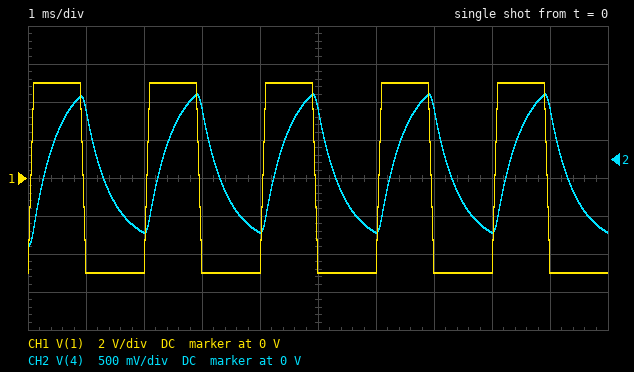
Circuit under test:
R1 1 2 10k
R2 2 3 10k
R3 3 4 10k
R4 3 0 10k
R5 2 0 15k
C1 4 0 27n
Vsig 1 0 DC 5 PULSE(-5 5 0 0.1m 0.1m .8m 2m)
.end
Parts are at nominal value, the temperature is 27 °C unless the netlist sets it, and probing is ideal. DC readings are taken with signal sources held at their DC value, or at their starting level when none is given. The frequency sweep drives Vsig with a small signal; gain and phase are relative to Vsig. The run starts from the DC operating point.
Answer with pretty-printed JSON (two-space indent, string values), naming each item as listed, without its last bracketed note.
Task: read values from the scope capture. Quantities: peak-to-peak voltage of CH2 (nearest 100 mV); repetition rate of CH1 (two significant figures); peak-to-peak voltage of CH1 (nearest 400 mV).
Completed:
{
  "peak-to-peak voltage of CH2": "2.0 V",
  "repetition rate of CH1": "500 Hz",
  "peak-to-peak voltage of CH1": "10.0 V"
}
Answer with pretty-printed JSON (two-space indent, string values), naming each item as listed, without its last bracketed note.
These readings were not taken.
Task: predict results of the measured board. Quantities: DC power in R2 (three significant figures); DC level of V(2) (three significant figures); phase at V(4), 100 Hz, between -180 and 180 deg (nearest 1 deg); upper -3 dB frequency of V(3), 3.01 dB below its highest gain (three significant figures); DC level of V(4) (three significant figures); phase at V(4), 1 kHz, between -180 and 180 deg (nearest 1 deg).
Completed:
{
  "DC power in R2": "133 µW",
  "DC level of V(2)": "2.31 V",
  "phase at V(4), 100 Hz, between -180 and 180 deg": "-15 deg",
  "upper -3 dB frequency of V(3), 3.01 dB below its highest gain": "755 Hz",
  "DC level of V(4)": "1.15 V",
  "phase at V(4), 1 kHz, between -180 and 180 deg": "-70 deg"
}
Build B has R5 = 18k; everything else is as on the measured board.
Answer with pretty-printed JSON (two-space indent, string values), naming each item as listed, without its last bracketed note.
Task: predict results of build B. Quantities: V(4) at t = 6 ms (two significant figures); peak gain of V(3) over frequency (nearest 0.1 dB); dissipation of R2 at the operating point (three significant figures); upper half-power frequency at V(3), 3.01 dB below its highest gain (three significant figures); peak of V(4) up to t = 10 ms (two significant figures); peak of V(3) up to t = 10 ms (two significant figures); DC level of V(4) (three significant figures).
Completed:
{
  "V(4) at t = 6 ms": "-1.0 V",
  "peak gain of V(3) over frequency": "-12.3 dB",
  "dissipation of R2 at the operating point": "148 µW",
  "upper half-power frequency at V(3), 3.01 dB below its highest gain": "743 Hz",
  "peak of V(4) up to t = 10 ms": "900 mV",
  "peak of V(3) up to t = 10 ms": "1.1 V",
  "DC level of V(4)": "1.22 V"
}
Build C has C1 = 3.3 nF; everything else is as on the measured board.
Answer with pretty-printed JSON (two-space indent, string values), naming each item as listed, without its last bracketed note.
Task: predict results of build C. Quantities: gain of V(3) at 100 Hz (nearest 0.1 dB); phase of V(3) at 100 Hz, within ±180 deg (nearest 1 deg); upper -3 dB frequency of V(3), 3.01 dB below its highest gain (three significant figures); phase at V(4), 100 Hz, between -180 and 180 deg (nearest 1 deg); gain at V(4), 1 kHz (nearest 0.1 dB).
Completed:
{
  "gain of V(3) at 100 Hz": "-12.7 dB",
  "phase of V(3) at 100 Hz, within ±180 deg": "-1 deg",
  "upper -3 dB frequency of V(3), 3.01 dB below its highest gain": "6.18 kHz",
  "phase at V(4), 100 Hz, between -180 and 180 deg": "-2 deg",
  "gain at V(4), 1 kHz": "-13.2 dB"
}
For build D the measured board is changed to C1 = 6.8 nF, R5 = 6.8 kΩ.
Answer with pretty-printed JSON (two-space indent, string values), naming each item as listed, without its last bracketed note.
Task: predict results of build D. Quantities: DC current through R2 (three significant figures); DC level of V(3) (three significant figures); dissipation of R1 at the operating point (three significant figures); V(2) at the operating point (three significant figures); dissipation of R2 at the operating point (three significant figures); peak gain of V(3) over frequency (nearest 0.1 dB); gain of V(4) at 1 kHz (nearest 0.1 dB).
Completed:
{
  "DC current through R2": "84.2 µA",
  "DC level of V(3)": "842 mV",
  "dissipation of R1 at the operating point": "1.10 mW",
  "V(2) at the operating point": "1.68 V",
  "dissipation of R2 at the operating point": "70.8 µW",
  "peak gain of V(3) over frequency": "-15.5 dB",
  "gain of V(4) at 1 kHz": "-17.1 dB"
}
